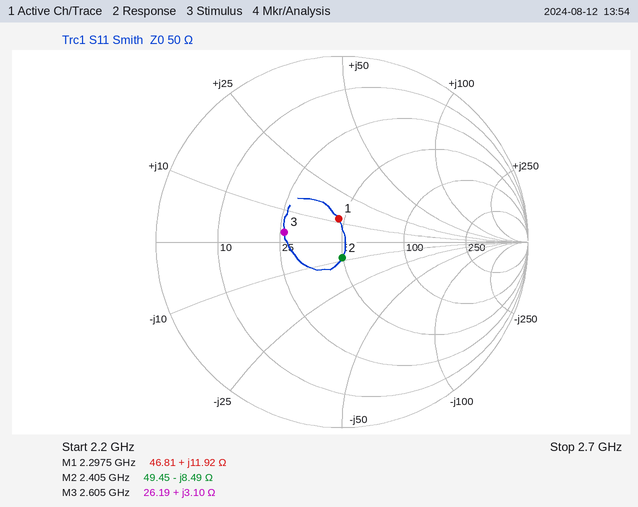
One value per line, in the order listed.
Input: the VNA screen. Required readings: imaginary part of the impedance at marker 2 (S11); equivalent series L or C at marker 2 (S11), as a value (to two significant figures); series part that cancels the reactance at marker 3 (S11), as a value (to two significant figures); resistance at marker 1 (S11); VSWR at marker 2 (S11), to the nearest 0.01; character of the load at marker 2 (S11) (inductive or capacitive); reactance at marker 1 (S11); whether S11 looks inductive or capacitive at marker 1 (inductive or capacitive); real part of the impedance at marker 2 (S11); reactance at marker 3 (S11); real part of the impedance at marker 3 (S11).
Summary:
-8.49 Ω
7.8 pF
20 pF
46.81 Ω
1.19
capacitive
+11.92 Ω
inductive
49.45 Ω
+3.10 Ω
26.19 Ω
